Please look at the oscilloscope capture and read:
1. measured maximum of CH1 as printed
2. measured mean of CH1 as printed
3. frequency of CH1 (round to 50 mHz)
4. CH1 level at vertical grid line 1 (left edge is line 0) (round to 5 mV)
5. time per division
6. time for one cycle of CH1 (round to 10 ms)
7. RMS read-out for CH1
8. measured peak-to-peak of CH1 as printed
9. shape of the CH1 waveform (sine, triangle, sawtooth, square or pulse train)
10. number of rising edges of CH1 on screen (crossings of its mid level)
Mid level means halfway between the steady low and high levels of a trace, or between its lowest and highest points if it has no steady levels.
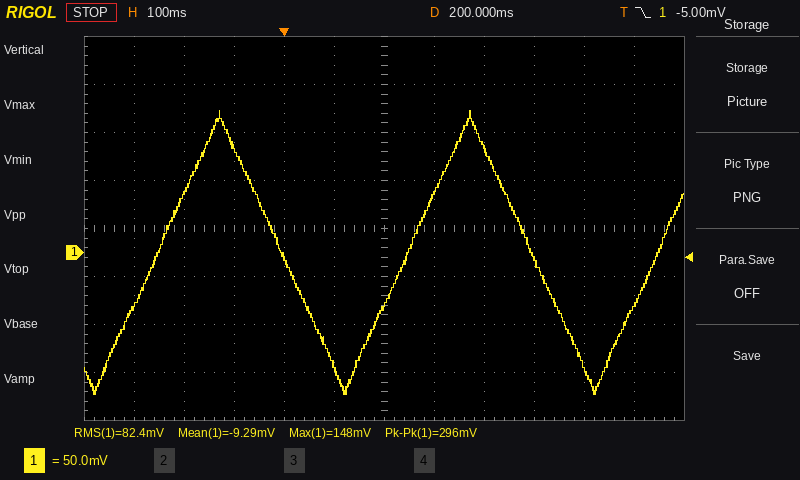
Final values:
148 mV
-9.29 mV
2.00 Hz
-55 mV
100 ms
500 ms
82.4 mV
296 mV
triangle
3
